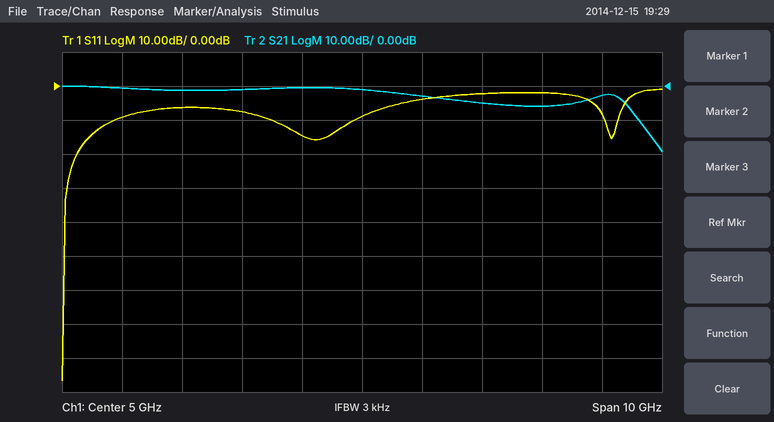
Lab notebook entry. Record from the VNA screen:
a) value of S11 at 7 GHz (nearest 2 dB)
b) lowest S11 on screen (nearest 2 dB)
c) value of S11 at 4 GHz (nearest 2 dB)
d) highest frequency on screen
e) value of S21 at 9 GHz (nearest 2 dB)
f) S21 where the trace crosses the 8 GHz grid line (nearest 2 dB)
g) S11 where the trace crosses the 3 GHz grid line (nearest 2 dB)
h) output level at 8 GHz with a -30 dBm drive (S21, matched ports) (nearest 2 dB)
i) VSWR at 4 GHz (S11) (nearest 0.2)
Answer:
-2 dB
-86 dB
-14 dB
10 GHz
-2 dB
-6 dB
-8 dB
-36 dBm
1.4
